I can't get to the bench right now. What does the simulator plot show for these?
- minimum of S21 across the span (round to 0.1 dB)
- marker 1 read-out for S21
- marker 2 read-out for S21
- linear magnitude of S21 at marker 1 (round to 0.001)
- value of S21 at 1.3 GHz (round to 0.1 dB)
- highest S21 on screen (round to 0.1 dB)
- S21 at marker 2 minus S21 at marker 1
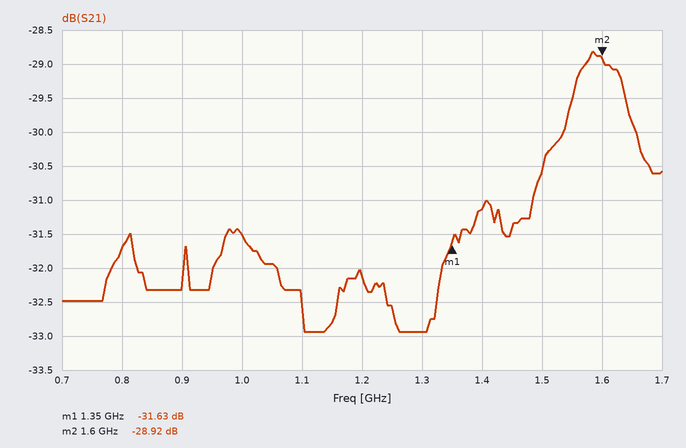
-32.9 dB
-31.63 dB
-28.92 dB
0.026
-32.9 dB
-28.8 dB
2.71 dB
